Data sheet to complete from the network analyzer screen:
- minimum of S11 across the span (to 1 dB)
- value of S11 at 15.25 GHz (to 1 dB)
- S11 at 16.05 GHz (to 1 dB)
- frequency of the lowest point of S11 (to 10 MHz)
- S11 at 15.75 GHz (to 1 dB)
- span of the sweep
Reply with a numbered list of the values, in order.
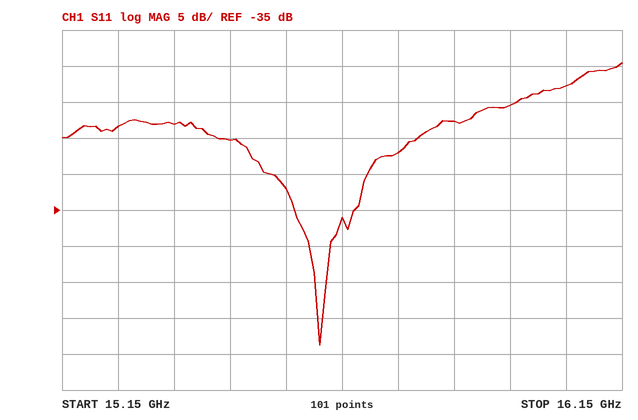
1. -54 dB
2. -23 dB
3. -18 dB
4. 15.61 GHz
5. -27 dB
6. 1 GHz
